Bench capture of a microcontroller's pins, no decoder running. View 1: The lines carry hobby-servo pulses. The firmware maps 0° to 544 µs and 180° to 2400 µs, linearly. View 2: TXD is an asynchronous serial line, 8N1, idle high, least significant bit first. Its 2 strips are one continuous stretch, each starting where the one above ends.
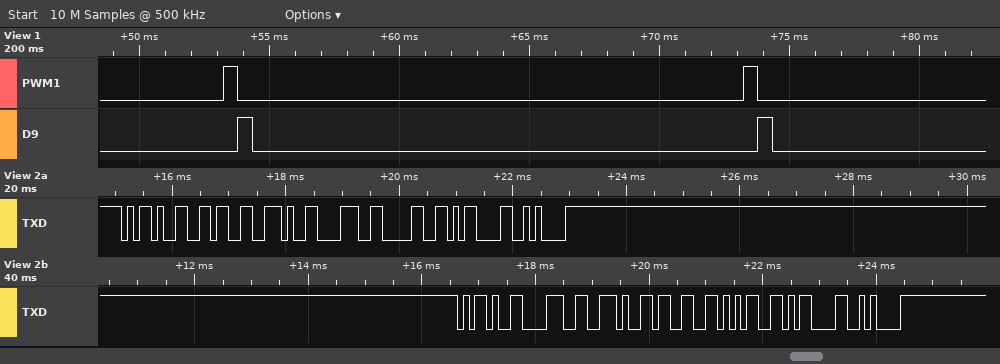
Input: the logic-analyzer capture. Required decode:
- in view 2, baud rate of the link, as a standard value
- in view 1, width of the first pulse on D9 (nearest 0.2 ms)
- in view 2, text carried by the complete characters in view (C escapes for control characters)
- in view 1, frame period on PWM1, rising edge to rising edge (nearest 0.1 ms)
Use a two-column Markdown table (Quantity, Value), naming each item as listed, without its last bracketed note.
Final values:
| Quantity | Value |
|---|---|
| in view 2, baud rate of the link, as a standard value | 9600 baud |
| in view 1, width of the first pulse on D9 | 0.6 ms |
| in view 2, text carried by the complete characters in view | "-6.80\r\n-8.35\r\n" |
| in view 1, frame period on PWM1, rising edge to rising edge | 20.0 ms |
